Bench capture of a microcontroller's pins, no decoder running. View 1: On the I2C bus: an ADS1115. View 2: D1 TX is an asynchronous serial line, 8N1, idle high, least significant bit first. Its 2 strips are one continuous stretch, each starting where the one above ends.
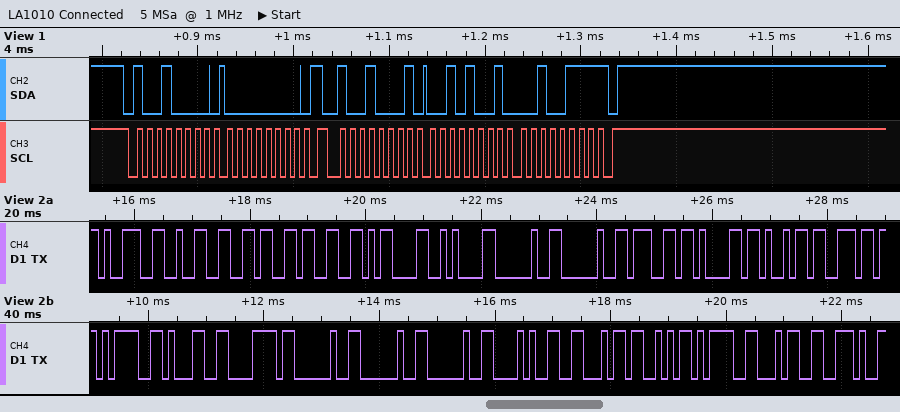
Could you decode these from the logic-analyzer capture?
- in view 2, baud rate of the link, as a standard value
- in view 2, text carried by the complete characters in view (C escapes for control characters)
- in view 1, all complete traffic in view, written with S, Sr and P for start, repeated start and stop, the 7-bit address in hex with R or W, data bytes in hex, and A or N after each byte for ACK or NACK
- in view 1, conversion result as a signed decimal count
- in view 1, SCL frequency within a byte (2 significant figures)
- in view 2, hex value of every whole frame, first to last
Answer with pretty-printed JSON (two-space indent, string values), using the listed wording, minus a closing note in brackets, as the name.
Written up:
{
  "in view 2, baud rate of the link, as a standard value": "9600 baud",
  "in view 2, text carried by the complete characters in view": "\"9263\\r\\n  gain=1x   (FS=4.\"",
  "in view 1, all complete traffic in view, written with S, Sr and P for start, repeated start and stop, the 7-bit address in hex with R or W, data bytes in hex, and A or N after each byte for ACK or NACK": "S 48W A 00 A Sr 48R A 29 A 27 N P",
  "in view 1, conversion result as a signed decimal count": "10535",
  "in view 1, SCL frequency within a byte": "100 kHz",
  "in view 2, hex value of every whole frame, first to last": "39 32 36 33 0D 0A 20 20 67 61 69 6E 3D 31 78 20 20 20 28 46 53 3D 34 2E"
}
